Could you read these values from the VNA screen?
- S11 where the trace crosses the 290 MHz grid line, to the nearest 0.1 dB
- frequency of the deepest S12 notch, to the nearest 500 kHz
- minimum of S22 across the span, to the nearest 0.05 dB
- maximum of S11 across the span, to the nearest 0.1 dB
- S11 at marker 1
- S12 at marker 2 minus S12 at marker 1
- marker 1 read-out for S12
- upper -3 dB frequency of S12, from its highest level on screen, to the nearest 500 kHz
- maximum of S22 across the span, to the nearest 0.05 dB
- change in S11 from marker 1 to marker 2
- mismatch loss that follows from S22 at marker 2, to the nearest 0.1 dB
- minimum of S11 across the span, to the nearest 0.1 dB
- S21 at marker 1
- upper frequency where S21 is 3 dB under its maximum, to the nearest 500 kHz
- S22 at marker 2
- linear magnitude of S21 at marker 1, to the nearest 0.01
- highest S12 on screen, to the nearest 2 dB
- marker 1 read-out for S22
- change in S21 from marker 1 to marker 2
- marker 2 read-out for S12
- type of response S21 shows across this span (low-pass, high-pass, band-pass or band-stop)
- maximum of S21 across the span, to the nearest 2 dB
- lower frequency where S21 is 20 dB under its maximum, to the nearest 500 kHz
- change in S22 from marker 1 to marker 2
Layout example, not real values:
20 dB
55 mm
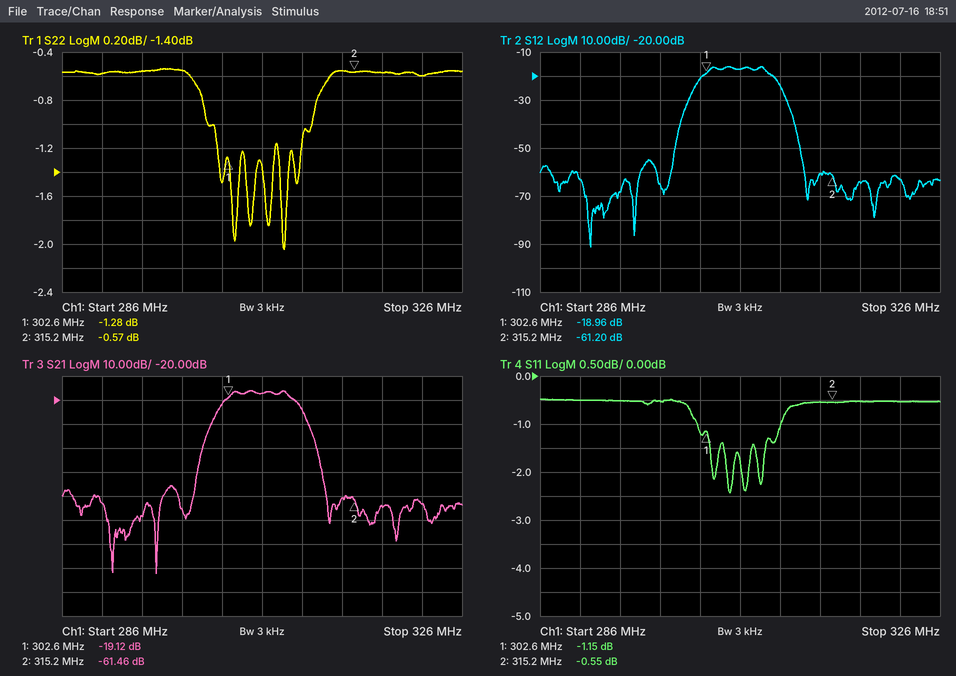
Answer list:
-0.5 dB
291.0 MHz
-2.05 dB
-0.5 dB
-1.15 dB
-42.24 dB
-18.96 dB
309.0 MHz
-0.55 dB
0.60 dB
9.1 dB
-2.4 dB
-19.12 dB
309.0 MHz
-0.57 dB
0.11
-16 dB
-1.28 dB
-42.34 dB
-61.20 dB
band-pass
-16 dB
300.5 MHz
0.71 dB
